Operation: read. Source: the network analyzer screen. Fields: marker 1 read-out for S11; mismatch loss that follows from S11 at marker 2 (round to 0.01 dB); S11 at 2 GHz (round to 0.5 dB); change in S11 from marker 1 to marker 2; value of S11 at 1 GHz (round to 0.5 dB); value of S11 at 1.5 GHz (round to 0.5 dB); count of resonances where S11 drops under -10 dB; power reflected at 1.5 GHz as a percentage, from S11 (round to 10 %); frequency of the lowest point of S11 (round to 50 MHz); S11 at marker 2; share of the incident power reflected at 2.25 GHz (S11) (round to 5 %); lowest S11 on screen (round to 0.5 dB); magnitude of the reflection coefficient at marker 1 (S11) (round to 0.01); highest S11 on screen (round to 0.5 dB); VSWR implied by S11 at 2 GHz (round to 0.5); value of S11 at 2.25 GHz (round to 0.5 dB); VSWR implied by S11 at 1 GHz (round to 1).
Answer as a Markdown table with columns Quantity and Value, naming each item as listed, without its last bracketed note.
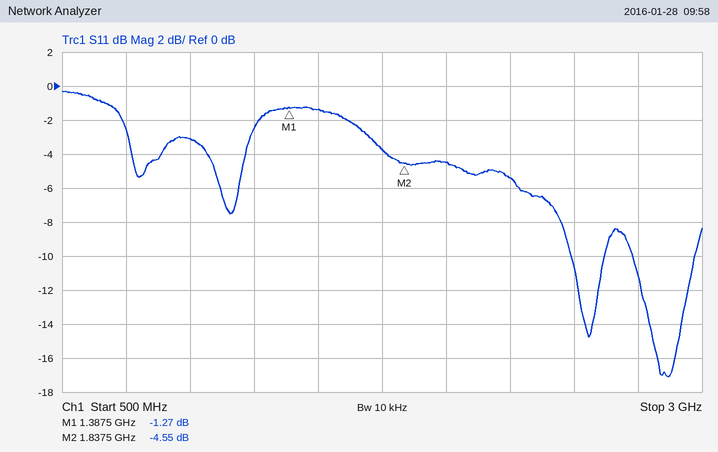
| Quantity | Value |
|---|---|
| marker 1 read-out for S11 | -1.27 dB |
| mismatch loss that follows from S11 at marker 2 | 1.88 dB |
| S11 at 2 GHz | -4.5 dB |
| change in S11 from marker 1 to marker 2 | -3.28 dB |
| value of S11 at 1 GHz | -3.0 dB |
| value of S11 at 1.5 GHz | -1.5 dB |
| count of resonances where S11 drops under -10 dB | 2 |
| power reflected at 1.5 GHz as a percentage, from S11 | 70 % |
| frequency of the lowest point of S11 | 2.85 GHz |
| S11 at marker 2 | -4.55 dB |
| share of the incident power reflected at 2.25 GHz (S11) | 30 % |
| lowest S11 on screen | -17.0 dB |
| magnitude of the reflection coefficient at marker 1 (S11) | 0.86 |
| highest S11 on screen | -0.5 dB |
| VSWR implied by S11 at 2 GHz | 4.0 |
| value of S11 at 2.25 GHz | -5.5 dB |
| VSWR implied by S11 at 1 GHz | 6 |
